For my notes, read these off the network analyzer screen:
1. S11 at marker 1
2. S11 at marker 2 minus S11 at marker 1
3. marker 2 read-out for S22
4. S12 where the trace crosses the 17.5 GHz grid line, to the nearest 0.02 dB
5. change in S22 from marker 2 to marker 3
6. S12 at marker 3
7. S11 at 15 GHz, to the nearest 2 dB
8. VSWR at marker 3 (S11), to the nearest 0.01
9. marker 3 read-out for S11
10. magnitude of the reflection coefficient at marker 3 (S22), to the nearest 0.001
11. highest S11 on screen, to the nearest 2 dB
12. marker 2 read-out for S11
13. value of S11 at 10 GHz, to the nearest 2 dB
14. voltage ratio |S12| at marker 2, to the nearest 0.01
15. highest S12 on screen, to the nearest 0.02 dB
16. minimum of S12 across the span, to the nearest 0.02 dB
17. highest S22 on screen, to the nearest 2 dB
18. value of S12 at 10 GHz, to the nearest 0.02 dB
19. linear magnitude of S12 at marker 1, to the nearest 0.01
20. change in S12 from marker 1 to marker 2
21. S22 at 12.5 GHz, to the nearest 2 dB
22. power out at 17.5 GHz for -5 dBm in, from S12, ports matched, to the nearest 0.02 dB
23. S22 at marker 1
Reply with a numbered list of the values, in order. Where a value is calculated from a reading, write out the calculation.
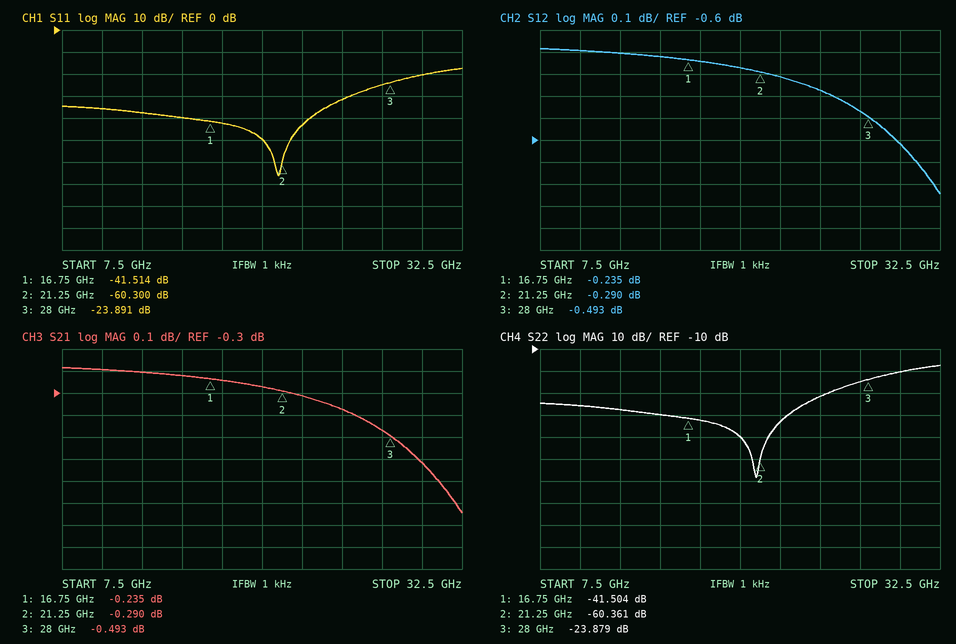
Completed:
1. -41.514 dB
2. -60.3 − (-41.514) = -18.786 dB
3. -60.361 dB
4. -0.24 dB
5. -23.879 − (-60.361) = 36.482 dB
6. -0.493 dB
7. -40 dB
8. (1 + 0.0639)/(1 − 0.0639) ≈ 1.14
9. -23.891 dB
10. 10^(-23.879/20) ≈ 0.064
11. -18 dB
12. -60.300 dB
13. -36 dB
14. 10^(-0.29/20) ≈ 0.97
15. -0.18 dB
16. -0.84 dB
17. -18 dB
18. -0.20 dB
19. 10^(-0.235/20) ≈ 0.97
20. -0.29 − (-0.235) = -0.055 dB
21. -38 dB
22. -5 dBm + (-0.24 dB) = -5.24 dBm
23. -41.504 dB
